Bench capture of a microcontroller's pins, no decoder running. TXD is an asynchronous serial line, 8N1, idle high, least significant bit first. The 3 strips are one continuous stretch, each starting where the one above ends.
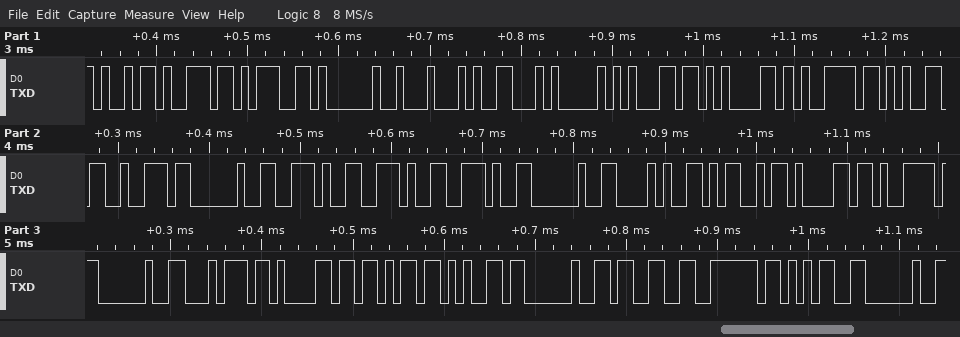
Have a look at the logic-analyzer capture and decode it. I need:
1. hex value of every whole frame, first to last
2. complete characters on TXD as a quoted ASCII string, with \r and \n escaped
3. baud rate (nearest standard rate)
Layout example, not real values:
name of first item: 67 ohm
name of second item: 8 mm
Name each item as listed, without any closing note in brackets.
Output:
hex value of every whole frame, first to last: 69 6E 67 20 44 46 50 6C 61 79 65 72 20 2E 2E 2E 20 28 4D 61 79 20 74 61 6B 65 20 33 7E 35 20
complete characters on TXD as a quoted ASCII string, with \r and \n escaped: "ing DFPlayer ... (May take 3~5 "
baud rate: 115200 baud
